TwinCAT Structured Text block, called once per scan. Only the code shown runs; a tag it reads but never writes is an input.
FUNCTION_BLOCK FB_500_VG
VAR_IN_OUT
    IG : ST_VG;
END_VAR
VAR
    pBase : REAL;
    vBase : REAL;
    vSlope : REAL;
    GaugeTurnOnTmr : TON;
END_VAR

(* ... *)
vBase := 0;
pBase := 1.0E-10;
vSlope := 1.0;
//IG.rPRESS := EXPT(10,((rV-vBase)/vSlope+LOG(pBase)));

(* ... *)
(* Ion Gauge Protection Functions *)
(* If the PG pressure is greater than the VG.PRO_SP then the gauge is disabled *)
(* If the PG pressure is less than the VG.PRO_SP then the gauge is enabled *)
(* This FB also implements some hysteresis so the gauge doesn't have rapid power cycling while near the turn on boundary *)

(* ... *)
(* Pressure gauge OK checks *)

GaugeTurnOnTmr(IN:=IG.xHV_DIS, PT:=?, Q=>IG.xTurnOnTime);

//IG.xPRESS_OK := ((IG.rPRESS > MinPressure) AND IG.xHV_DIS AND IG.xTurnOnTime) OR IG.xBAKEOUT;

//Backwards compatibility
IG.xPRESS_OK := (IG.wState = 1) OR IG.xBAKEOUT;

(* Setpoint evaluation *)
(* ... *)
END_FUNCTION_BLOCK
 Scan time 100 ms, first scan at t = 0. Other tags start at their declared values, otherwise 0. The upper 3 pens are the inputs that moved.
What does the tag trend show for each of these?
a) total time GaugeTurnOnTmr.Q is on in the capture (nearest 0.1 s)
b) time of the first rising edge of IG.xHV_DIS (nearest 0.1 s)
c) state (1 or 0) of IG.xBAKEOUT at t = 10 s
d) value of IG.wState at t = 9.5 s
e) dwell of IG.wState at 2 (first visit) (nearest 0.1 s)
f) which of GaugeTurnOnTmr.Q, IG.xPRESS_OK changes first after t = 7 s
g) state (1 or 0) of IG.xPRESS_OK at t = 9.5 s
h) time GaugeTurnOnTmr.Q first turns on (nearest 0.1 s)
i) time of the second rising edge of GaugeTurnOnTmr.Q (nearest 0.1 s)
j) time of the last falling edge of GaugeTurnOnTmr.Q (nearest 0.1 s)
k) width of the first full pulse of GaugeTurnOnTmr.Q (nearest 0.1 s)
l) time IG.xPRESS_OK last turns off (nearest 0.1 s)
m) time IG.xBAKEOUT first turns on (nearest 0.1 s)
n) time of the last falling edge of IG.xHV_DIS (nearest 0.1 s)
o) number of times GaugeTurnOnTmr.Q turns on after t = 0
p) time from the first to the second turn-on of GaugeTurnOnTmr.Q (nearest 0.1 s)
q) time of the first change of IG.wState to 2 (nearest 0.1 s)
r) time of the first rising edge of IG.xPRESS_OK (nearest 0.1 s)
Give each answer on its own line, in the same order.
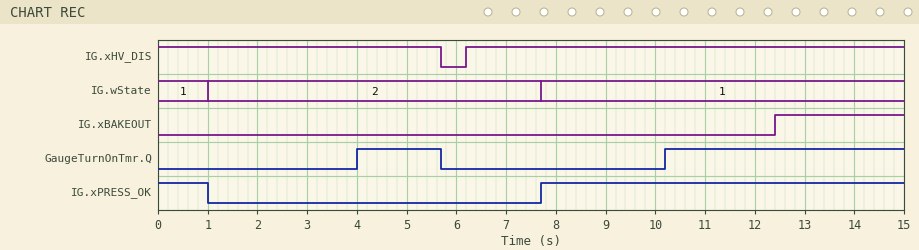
6.5 s
6.2 s
0
1
6.7 s
IG.xPRESS_OK
1
4.0 s
10.2 s
5.7 s
1.7 s
1.0 s
12.4 s
5.7 s
2
6.2 s
1.0 s
7.7 s
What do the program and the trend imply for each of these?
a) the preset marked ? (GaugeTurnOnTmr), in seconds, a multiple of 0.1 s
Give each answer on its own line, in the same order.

4.0 s
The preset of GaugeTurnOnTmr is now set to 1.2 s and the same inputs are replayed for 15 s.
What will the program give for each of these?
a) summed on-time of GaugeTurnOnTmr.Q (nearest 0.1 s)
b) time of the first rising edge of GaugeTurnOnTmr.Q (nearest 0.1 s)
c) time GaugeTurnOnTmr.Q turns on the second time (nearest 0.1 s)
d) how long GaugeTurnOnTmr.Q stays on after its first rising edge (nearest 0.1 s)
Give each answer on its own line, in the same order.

12.1 s
1.2 s
7.4 s
4.5 s
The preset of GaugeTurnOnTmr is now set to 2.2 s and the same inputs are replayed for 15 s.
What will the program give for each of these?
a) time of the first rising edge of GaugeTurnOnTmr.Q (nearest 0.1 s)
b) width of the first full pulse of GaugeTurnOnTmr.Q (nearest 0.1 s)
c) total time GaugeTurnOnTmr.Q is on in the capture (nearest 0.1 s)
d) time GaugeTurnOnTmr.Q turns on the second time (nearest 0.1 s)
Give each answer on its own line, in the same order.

2.2 s
3.5 s
10.1 s
8.4 s
